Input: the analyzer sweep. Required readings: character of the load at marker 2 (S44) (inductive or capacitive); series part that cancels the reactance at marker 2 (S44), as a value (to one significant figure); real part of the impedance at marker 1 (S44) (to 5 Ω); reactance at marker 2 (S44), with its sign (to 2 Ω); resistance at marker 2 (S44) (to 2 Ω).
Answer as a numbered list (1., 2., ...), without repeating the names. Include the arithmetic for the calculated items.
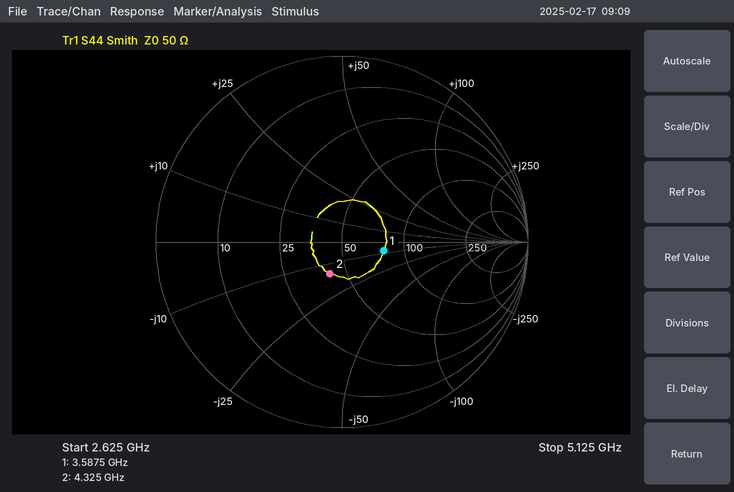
1. capacitive
2. L = 14 Ω/(2π × 4.325 GHz) ≈ 515 pH, so 500 pH to one significant figure
3. 80 Ω
4. -14 Ω
5. 42 Ω
